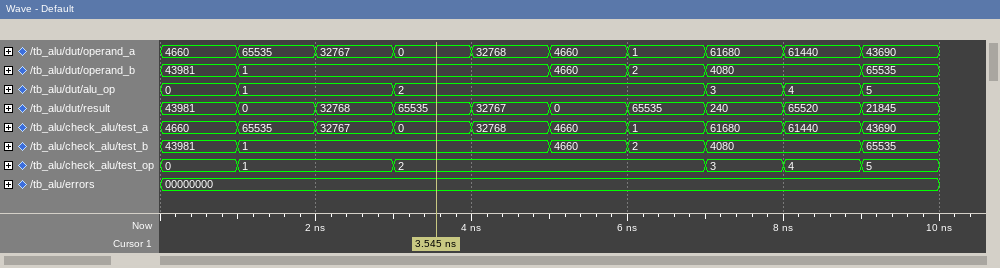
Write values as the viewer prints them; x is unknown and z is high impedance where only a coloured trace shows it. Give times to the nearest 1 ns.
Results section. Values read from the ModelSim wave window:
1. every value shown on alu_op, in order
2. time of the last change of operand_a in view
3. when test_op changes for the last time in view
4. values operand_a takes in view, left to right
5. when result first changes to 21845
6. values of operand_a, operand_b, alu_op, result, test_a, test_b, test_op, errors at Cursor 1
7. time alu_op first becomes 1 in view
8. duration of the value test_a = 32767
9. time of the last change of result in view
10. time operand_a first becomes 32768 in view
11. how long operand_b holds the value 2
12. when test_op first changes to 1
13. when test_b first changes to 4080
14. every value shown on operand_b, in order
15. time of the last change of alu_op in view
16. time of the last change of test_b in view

0, 1, 2, 3, 4, 5
9 ns
9 ns
4660, 65535, 32767, 0, 32768, 4660, 1, 61680, 61440, 43690
9 ns
operand_a=0, operand_b=1, alu_op=2, result=65535, test_a=0, test_b=1, test_op=2, errors=00000000
1 ns
1 ns
9 ns
4 ns
1 ns
1 ns
7 ns
43981, 1, 4660, 2, 4080, 65535
9 ns
9 ns
